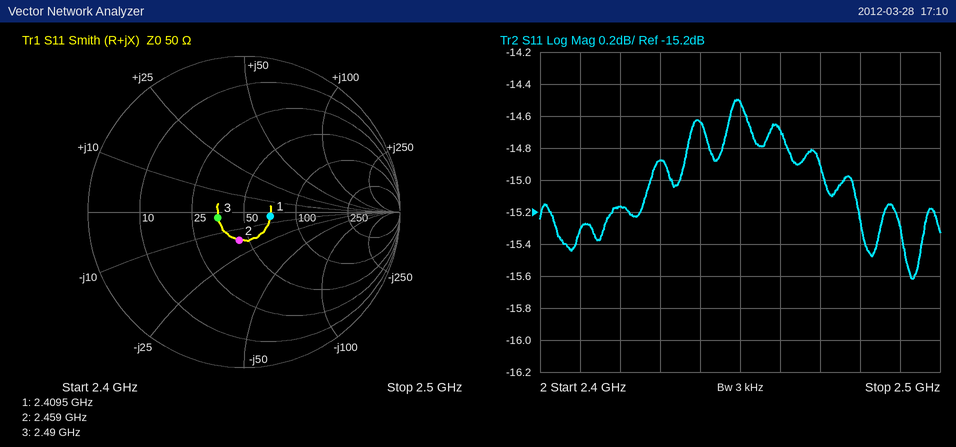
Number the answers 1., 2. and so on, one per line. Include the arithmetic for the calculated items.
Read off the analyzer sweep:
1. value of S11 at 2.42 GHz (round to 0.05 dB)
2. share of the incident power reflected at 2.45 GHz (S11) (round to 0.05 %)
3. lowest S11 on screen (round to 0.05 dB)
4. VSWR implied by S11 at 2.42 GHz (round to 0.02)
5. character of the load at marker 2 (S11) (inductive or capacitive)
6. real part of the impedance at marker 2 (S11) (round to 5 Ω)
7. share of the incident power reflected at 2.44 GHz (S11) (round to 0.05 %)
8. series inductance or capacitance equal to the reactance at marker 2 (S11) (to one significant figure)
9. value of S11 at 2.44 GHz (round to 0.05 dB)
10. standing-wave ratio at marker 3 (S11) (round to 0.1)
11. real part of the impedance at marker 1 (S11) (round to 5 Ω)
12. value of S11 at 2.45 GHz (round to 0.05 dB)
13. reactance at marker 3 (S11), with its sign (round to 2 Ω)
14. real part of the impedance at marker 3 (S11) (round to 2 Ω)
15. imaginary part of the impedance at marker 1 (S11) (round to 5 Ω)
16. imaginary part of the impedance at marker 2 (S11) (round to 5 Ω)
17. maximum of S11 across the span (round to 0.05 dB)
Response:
1. -15.15 dB
2. 10^(-14.5/10) ≈ 3.55 %
3. -15.60 dB
4. |Γ| = 10^(-15.15/20) = 0.1748; VSWR = (1 + 0.1748)/(1 − 0.1748) ≈ 1.42
5. capacitive
6. 45 Ω
7. 10^(-14.65/10) ≈ 3.43 %, so 3.45 % to the nearest 0.05 %
8. C = 1/(2π × 2.459 GHz × 15 Ω) ≈ 4 pF
9. -14.65 dB
10. 1.4
11. 70 Ω
12. -14.50 dB
13. -2 Ω
14. 36 Ω
15. -5 Ω
16. -15 Ω
17. -14.50 dB
